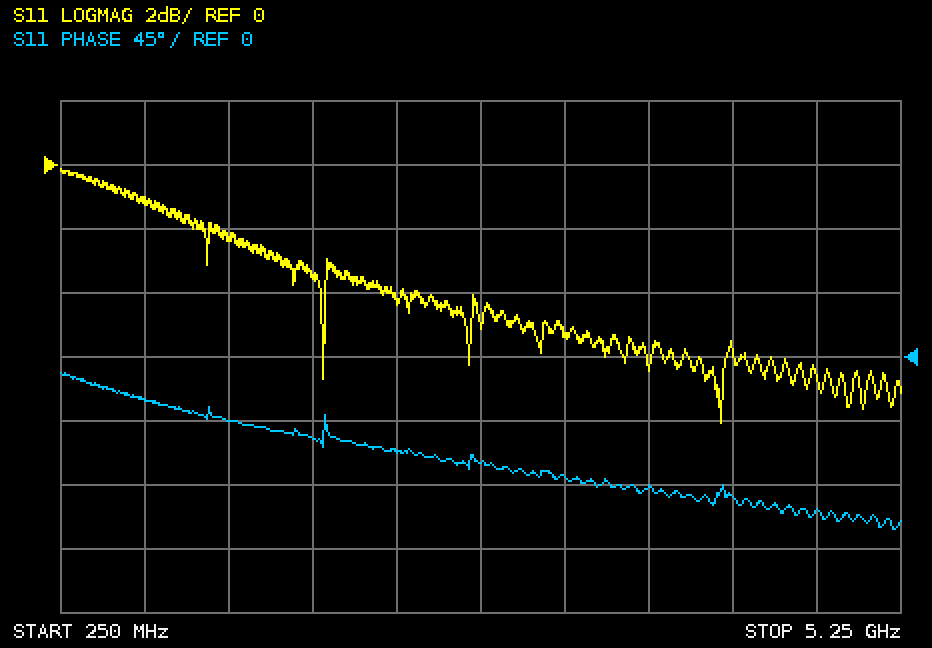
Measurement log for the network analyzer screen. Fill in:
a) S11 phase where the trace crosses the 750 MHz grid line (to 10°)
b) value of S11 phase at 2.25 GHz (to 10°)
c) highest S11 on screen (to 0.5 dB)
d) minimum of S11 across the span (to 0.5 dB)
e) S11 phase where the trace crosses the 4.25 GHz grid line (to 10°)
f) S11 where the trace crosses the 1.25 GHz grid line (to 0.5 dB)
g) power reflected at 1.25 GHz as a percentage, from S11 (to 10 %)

-30°
-70°
0.0 dB
-8.0 dB
-100°
-2.5 dB
60 %
